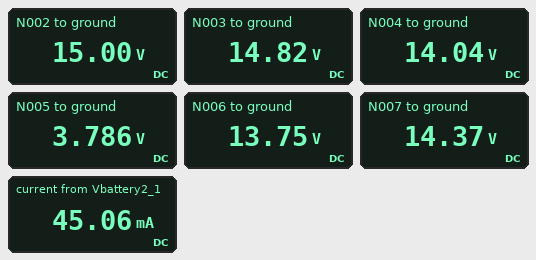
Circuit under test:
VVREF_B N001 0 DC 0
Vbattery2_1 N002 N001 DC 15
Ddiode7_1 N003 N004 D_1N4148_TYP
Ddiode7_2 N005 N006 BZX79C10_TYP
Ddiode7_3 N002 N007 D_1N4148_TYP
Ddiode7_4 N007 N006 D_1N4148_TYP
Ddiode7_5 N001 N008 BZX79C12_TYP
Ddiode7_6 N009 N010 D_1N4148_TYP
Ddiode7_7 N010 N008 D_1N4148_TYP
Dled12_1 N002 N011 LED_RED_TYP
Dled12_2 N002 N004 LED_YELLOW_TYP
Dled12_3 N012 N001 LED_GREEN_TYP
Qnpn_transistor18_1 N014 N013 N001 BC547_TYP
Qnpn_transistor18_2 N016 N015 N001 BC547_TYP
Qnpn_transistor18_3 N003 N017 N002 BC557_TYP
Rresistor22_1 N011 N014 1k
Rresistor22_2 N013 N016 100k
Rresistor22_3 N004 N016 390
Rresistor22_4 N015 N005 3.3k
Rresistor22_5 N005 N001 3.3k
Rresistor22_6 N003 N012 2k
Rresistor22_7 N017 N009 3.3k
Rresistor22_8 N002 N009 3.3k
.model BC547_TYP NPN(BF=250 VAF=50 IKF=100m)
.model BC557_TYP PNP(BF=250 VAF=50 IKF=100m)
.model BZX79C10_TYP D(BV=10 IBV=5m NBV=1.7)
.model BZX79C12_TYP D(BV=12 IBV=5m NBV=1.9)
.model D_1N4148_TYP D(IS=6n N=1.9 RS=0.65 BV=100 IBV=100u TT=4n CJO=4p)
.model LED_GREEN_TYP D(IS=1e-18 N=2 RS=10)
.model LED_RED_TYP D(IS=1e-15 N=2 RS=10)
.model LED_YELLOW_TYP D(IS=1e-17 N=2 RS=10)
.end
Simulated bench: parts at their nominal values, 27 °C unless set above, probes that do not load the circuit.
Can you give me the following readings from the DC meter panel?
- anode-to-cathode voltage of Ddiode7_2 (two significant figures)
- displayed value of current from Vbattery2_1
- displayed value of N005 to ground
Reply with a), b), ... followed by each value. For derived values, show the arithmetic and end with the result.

a) 3.786 V - 13.75 V = -10 V
b) 45.06 mA
c) 3.786 V
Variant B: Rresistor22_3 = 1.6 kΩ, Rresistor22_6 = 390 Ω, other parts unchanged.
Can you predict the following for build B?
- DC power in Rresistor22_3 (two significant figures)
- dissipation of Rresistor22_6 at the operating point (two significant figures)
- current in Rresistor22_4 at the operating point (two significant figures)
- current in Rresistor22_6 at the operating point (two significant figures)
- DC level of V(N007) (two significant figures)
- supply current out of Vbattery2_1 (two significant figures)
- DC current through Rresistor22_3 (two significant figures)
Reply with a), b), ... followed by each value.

a) 120 mW
b) 400 mW
c) 890 µA
d) 32 mA
e) 14 V
f) 44 mA
g) 8.8 mA
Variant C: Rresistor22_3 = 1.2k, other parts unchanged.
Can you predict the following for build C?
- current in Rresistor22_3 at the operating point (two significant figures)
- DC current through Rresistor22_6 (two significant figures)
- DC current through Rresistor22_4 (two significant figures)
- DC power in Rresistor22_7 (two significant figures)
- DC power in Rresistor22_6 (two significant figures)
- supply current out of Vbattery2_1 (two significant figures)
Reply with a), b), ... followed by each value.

a) 12 mA
b) 6.5 mA
c) 890 µA
d) 340 µW
e) 84 mW
f) 21 mA
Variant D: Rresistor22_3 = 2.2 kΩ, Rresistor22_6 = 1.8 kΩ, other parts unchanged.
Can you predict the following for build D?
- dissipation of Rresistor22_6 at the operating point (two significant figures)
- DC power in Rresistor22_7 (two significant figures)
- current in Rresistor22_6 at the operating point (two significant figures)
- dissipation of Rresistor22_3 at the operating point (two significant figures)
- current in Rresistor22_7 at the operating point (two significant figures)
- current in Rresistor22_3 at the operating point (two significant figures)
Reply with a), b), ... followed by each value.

a) 93 mW
b) 340 µW
c) 7.2 mA
d) 91 mW
e) 320 µA
f) 6.4 mA
